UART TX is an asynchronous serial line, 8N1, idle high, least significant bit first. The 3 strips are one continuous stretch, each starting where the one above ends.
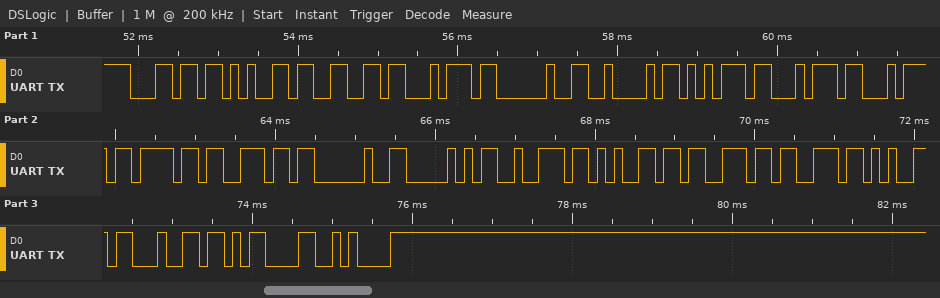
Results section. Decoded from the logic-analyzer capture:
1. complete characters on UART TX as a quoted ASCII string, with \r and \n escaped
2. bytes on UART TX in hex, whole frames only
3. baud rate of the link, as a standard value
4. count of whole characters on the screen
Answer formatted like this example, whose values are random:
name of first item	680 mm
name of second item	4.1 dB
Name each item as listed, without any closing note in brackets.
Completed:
complete characters on UART TX as a quoted ASCII string, with \r and \n escaped	"left Button Pressed\r\n"
bytes on UART TX in hex, whole frames only	0x6C 0x65 0x66 0x74 0x20 0x42 0x75 0x74 0x74 0x6F 0x6E 0x20 0x50 0x72 0x65 0x73 0x73 0x65 0x64 0x0D 0x0A
baud rate of the link, as a standard value	9600 baud
count of whole characters on the screen	21
